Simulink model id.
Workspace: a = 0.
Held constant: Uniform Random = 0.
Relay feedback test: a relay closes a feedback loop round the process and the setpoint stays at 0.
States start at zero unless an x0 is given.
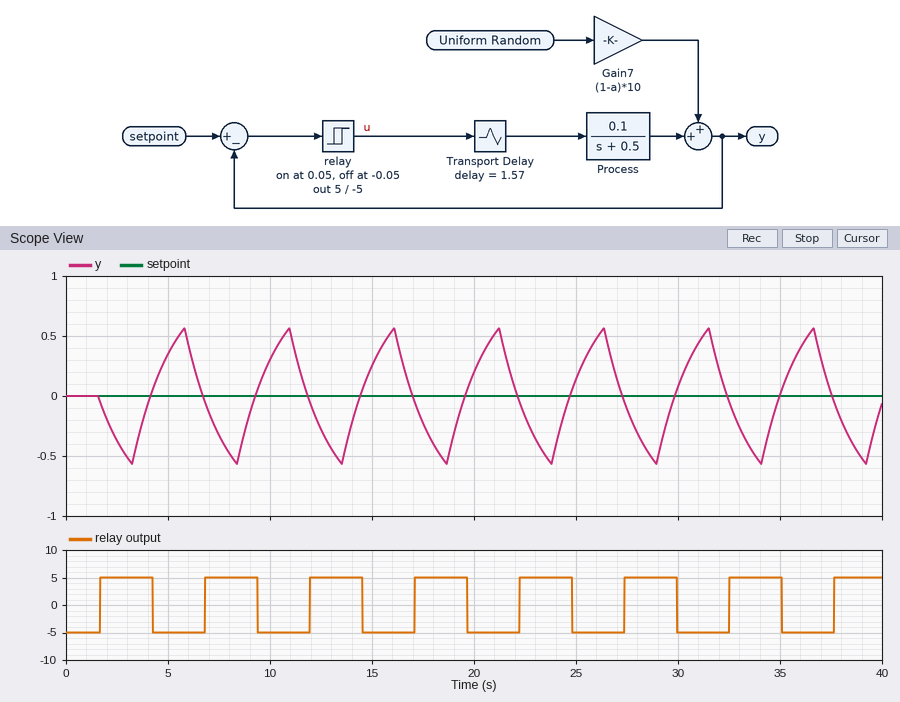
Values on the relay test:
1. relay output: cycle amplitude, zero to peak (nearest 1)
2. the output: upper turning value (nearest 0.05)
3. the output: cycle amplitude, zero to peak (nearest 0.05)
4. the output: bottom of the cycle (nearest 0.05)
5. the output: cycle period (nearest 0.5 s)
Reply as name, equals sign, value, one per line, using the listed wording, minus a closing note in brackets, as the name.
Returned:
relay output: cycle amplitude, zero to peak = 5
the output: upper turning value = 0.55
the output: cycle amplitude, zero to peak = 0.55
the output: bottom of the cycle = -0.55
the output: cycle period = 5.0 s
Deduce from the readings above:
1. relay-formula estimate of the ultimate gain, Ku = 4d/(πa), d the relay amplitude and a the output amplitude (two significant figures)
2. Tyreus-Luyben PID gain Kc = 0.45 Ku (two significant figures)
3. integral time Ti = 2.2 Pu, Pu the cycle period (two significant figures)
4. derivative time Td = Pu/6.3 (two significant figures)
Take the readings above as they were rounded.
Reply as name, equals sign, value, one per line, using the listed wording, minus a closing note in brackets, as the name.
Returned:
relay-formula estimate of the ultimate gain, Ku = 4d/(πa), d the relay amplitude and a the output amplitude = 12
Tyreus-Luyben PID gain Kc = 0.45 Ku = 5.4
integral time Ti = 2.2 Pu, Pu the cycle period = 11 s
derivative time Td = Pu/6.3 = 0.79 s
